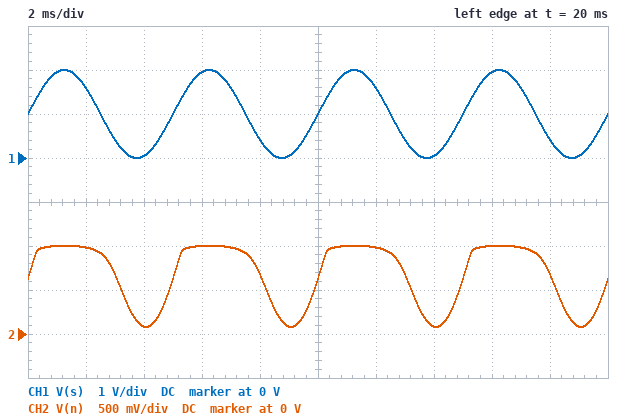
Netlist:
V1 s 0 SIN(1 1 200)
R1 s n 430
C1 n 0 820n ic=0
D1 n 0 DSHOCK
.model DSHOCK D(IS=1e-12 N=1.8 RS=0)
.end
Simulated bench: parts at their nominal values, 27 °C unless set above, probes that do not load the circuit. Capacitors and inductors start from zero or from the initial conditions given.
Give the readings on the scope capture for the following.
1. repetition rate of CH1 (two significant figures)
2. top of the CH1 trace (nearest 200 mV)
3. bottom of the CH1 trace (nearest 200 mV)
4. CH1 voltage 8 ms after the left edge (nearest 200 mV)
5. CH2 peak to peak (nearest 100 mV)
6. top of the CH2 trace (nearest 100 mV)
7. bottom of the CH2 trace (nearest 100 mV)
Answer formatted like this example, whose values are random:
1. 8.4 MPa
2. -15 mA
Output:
1. 200 Hz
2. 2.0 V
3. 0 V
4. 400 mV
5. 900 mV
6. 1.0 V
7. 100 mV
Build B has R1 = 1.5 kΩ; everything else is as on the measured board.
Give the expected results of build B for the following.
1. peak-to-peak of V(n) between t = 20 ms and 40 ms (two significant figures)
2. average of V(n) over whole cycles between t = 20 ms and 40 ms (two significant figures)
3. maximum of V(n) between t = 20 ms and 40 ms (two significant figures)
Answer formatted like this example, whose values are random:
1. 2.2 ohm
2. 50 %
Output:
1. 620 mV
2. 700 mV
3. 950 mV
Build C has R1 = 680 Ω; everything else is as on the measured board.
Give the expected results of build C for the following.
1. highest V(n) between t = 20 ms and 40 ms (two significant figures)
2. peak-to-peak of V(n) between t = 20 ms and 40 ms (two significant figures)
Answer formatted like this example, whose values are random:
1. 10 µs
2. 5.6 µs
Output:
1. 980 mV
2. 830 mV
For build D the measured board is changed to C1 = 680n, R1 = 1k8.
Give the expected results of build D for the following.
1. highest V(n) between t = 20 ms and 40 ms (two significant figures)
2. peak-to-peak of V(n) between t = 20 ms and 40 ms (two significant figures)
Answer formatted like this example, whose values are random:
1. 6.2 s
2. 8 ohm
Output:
1. 940 mV
2. 610 mV
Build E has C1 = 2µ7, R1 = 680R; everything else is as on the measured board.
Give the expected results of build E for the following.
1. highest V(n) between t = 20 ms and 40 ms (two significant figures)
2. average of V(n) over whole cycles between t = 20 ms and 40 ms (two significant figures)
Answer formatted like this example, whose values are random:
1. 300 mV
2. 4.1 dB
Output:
1. 980 mV
2. 750 mV
